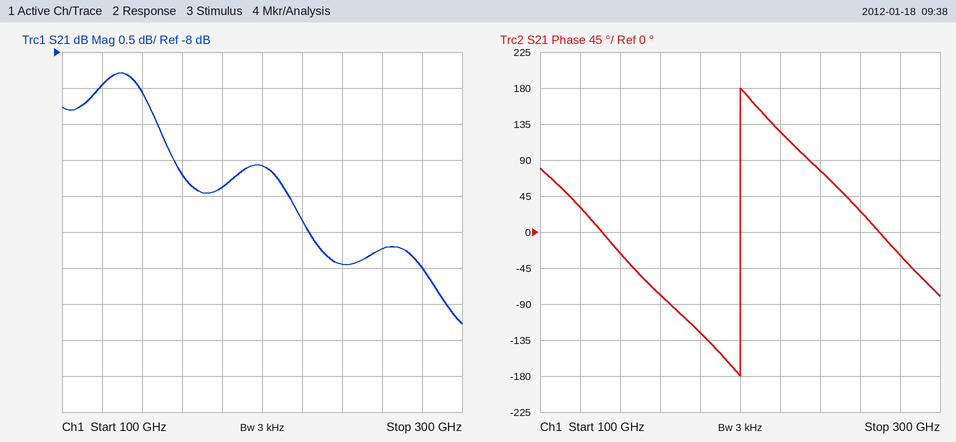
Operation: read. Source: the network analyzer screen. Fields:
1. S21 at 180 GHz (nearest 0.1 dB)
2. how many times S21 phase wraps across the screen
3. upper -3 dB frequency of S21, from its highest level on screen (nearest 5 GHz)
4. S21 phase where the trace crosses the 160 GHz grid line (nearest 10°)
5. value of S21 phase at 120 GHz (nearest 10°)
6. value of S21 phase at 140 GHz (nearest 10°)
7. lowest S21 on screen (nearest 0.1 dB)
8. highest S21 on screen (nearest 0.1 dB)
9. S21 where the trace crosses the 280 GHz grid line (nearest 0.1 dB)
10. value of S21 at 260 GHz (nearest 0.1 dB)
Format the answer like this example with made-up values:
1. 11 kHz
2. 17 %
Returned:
1. -9.9 dB
2. 1
3. 285 GHz
4. -80°
5. 30°
6. -30°
7. -11.8 dB
8. -8.3 dB
9. -11.0 dB
10. -10.7 dB
